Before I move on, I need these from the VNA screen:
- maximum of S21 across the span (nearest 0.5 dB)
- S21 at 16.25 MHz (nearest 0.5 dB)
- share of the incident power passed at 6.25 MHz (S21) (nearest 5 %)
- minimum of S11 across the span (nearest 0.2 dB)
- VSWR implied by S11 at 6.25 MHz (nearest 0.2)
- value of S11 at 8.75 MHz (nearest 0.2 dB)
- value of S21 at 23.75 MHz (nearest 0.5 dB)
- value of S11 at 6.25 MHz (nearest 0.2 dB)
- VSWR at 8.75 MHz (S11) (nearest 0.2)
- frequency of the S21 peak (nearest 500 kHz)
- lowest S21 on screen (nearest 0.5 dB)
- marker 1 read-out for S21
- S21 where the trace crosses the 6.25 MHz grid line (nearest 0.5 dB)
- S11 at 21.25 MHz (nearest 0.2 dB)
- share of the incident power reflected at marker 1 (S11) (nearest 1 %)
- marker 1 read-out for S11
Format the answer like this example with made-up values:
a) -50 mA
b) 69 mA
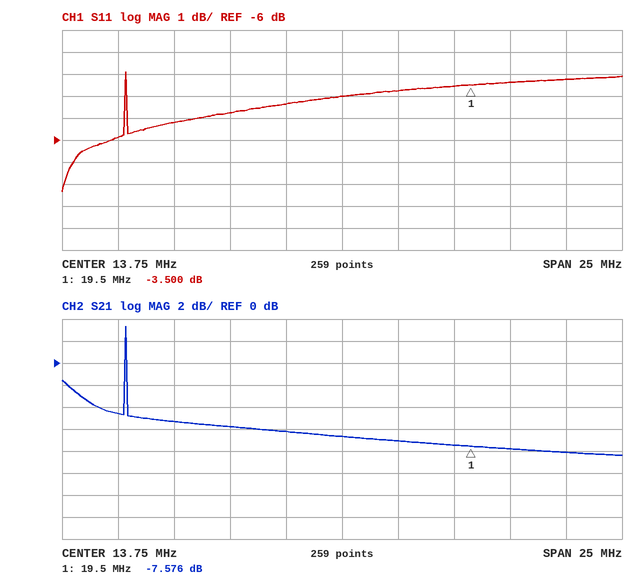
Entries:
a) 3.5 dB
b) -7.0 dB
c) 30 %
d) -8.4 dB
e) 3.4
f) -4.8 dB
g) -8.0 dB
h) -5.2 dB
i) 3.8
j) 4.0 MHz
k) -8.5 dB
l) -7.576 dB
m) -5.5 dB
n) -3.4 dB
o) 45 %
p) -3.500 dB
